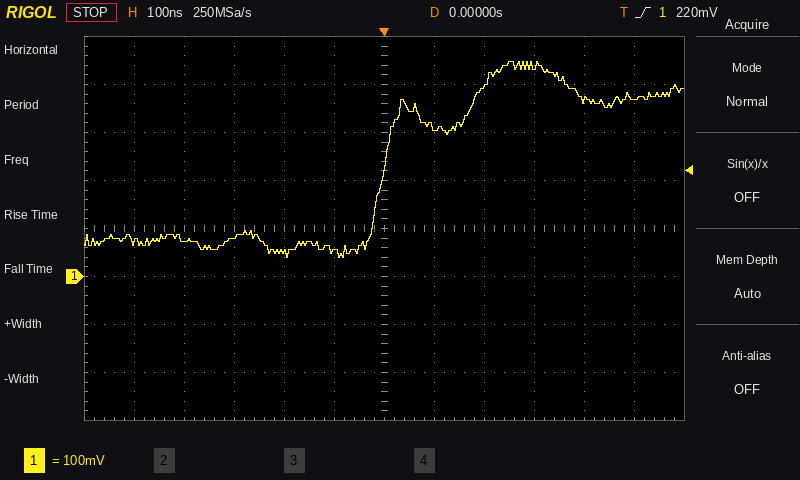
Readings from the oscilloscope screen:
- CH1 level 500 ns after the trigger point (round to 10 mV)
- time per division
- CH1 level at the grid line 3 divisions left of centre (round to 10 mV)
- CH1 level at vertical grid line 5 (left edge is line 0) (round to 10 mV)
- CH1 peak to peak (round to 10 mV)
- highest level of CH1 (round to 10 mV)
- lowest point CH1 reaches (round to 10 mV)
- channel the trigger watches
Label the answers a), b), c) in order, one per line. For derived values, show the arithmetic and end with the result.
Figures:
a) 370 mV
b) 100 ns
c) 80 mV
d) 50 mV
e) 450 mV − (40 mV) = 410 mV
f) 450 mV
g) 40 mV
h) CH1
